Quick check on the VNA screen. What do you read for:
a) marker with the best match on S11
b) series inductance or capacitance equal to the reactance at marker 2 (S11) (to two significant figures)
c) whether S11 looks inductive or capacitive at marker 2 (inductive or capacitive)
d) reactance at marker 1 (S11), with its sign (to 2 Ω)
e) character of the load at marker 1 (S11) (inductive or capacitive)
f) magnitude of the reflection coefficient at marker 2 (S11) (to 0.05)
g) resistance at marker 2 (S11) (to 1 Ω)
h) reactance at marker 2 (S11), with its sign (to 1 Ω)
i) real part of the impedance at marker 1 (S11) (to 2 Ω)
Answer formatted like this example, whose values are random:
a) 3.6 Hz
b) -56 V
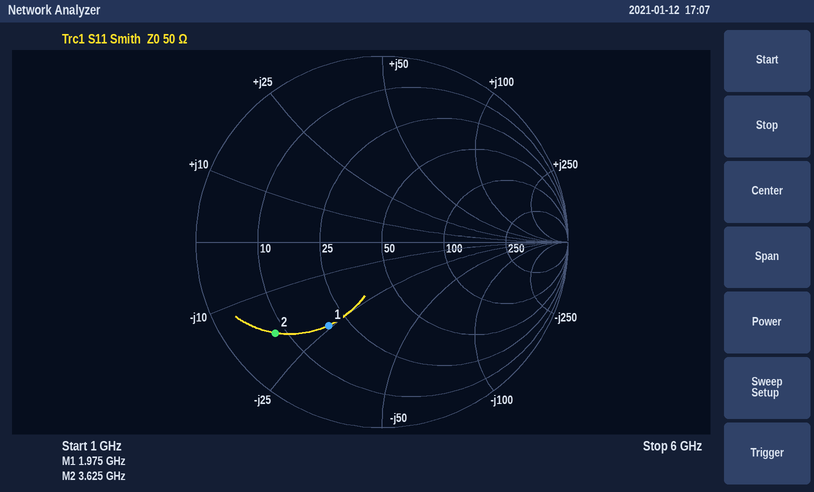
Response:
a) marker 1
b) 2.4 pF
c) capacitive
d) -24 Ω
e) capacitive
f) 0.75
g) 8 Ω
h) -18 Ω
i) 20 Ω
